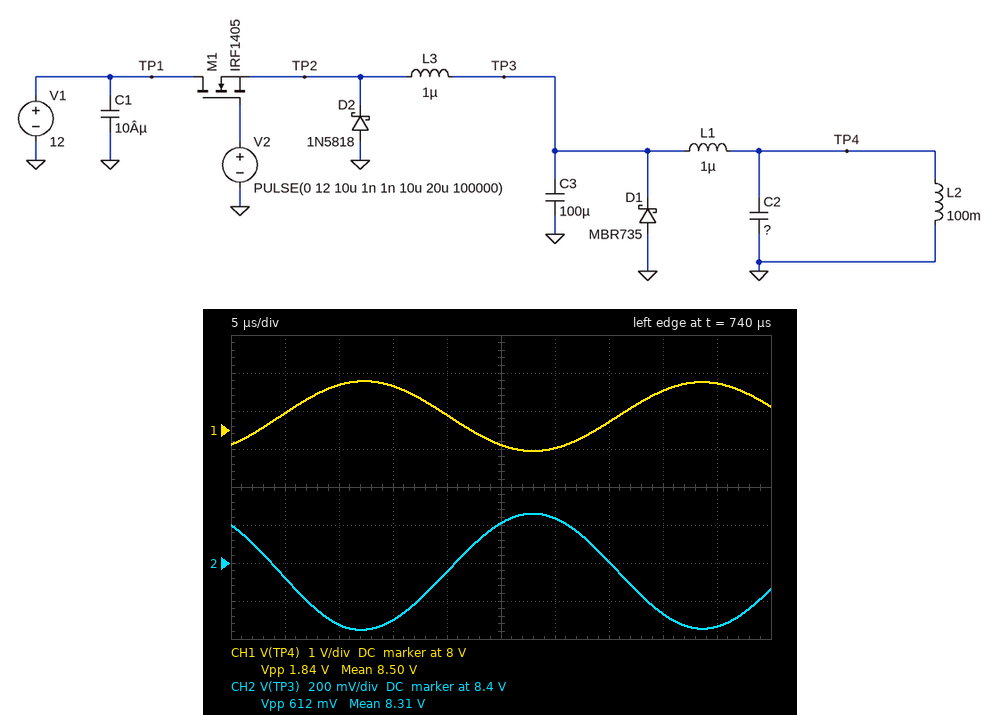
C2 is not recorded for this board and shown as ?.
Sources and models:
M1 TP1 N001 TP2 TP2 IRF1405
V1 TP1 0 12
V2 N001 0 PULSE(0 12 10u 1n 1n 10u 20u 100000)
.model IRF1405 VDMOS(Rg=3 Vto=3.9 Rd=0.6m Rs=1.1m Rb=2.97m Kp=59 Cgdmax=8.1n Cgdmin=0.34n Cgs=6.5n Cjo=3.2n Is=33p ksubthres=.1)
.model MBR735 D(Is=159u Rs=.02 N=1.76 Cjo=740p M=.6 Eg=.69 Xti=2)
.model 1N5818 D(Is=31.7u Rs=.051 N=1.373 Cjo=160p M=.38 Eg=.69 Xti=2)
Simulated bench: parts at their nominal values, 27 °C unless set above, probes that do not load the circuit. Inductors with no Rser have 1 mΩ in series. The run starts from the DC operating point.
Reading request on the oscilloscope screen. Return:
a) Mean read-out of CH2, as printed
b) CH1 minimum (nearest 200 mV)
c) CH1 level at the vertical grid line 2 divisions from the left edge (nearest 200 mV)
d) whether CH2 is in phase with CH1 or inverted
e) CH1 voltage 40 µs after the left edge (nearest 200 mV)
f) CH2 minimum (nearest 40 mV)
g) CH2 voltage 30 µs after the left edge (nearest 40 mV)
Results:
8.31 V
7.4 V
9.2 V
inverted
9.0 V
8.04 V
8.64 V
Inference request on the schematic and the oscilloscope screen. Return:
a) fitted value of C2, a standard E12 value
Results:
33 µF
